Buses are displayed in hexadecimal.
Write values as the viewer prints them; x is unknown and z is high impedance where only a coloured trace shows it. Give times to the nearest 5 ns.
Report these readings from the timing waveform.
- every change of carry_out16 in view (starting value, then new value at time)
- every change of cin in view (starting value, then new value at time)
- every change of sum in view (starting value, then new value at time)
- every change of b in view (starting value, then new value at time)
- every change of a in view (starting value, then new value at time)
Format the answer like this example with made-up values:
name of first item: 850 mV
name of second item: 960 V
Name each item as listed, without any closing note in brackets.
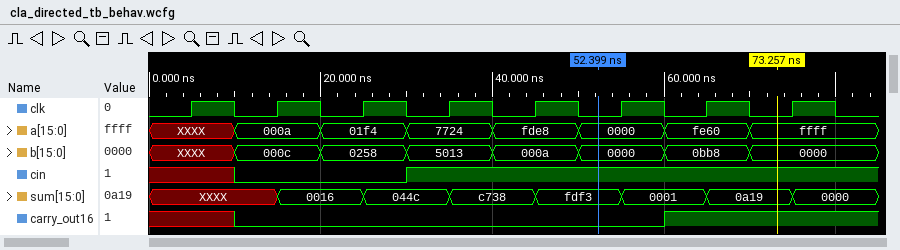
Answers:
every change of carry_out16 in view: x, 0 at 10 ns, 1 at 60 ns
every change of cin in view: x, 0 at 10 ns, 1 at 30 ns
every change of sum in view: XXXX, 0016 at 15 ns, 044c at 25 ns, c738 at 35 ns, fdf3 at 45 ns, 0001 at 55 ns, 0a19 at 65 ns, 0000 at 75 ns
every change of b in view: XXXX, 000c at 10 ns, 0258 at 20 ns, 5013 at 30 ns, 000a at 40 ns, 0000 at 50 ns, 0bb8 at 60 ns, 0000 at 70 ns
every change of a in view: XXXX, 000a at 10 ns, 01f4 at 20 ns, 7724 at 30 ns, fde8 at 40 ns, 0000 at 50 ns, fe60 at 60 ns, ffff at 70 ns
